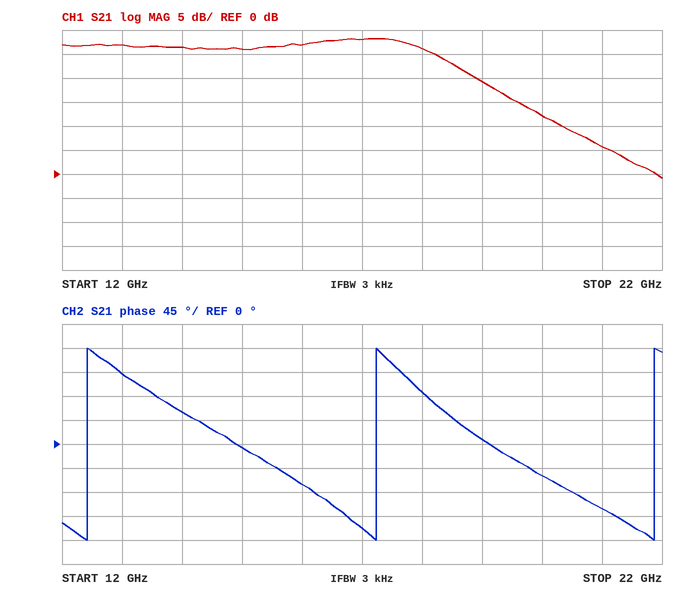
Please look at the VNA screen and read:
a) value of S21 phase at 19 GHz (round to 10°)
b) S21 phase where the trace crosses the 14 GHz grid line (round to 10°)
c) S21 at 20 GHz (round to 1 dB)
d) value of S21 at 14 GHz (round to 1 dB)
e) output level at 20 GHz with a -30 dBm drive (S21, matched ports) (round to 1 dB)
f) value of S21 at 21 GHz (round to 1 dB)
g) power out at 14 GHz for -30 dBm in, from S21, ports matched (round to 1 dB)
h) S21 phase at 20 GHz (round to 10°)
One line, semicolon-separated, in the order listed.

10°; 60°; 12 dB; 26 dB; -18 dBm; 6 dB; -4 dBm; -60°
